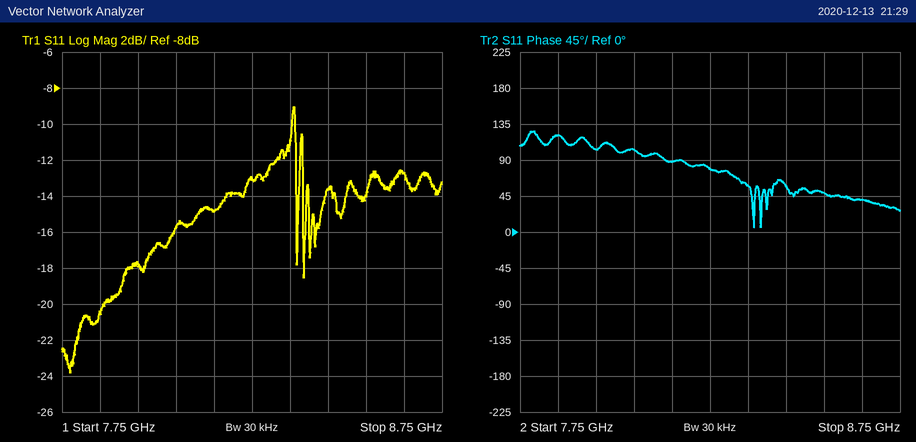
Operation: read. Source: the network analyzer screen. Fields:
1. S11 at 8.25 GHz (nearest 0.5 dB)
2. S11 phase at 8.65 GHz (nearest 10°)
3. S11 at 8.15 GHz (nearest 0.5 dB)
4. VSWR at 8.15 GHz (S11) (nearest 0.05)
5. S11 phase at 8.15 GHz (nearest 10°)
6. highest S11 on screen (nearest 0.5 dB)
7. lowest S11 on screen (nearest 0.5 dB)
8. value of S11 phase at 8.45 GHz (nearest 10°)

-13.0 dB
40°
-15.0 dB
1.45
90°
-9.0 dB
-24.0 dB
60°
